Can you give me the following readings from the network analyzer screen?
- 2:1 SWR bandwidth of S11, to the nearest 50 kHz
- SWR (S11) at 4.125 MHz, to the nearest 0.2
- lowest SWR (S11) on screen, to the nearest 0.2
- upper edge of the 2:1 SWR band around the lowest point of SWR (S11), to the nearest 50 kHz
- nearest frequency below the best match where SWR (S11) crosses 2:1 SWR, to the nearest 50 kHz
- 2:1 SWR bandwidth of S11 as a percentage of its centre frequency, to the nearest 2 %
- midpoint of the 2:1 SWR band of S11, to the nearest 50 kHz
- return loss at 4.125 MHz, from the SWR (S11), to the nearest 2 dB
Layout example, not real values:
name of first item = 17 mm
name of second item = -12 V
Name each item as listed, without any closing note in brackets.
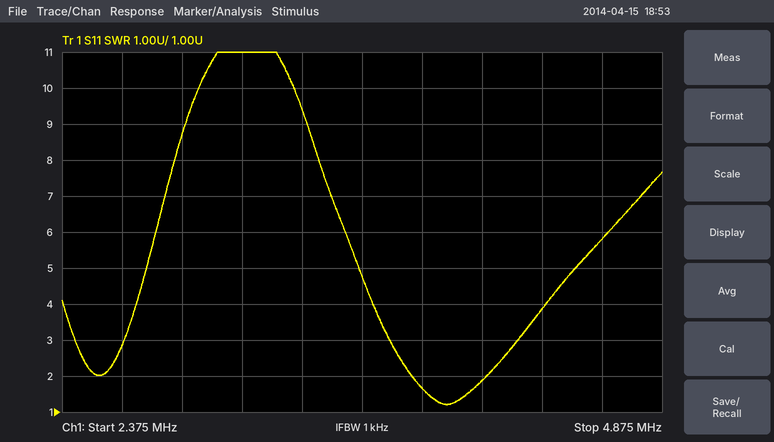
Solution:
2:1 SWR bandwidth of S11, to the nearest 50 kHz = 300 kHz
SWR (S11) at 4.125 MHz, to the nearest 0.2 = 1.8
lowest SWR (S11) on screen, to the nearest 0.2 = 1.2
upper edge of the 2:1 SWR band around the lowest point of SWR (S11), to the nearest 50 kHz = 4.15 MHz
nearest frequency below the best match where SWR (S11) crosses 2:1 SWR, to the nearest 50 kHz = 3.85 MHz
2:1 SWR bandwidth of S11 as a percentage of its centre frequency, to the nearest 2 % = 8 %
midpoint of the 2:1 SWR band of S11, to the nearest 50 kHz = 4.00 MHz
return loss at 4.125 MHz, from the SWR (S11), to the nearest 2 dB = 10 dB
